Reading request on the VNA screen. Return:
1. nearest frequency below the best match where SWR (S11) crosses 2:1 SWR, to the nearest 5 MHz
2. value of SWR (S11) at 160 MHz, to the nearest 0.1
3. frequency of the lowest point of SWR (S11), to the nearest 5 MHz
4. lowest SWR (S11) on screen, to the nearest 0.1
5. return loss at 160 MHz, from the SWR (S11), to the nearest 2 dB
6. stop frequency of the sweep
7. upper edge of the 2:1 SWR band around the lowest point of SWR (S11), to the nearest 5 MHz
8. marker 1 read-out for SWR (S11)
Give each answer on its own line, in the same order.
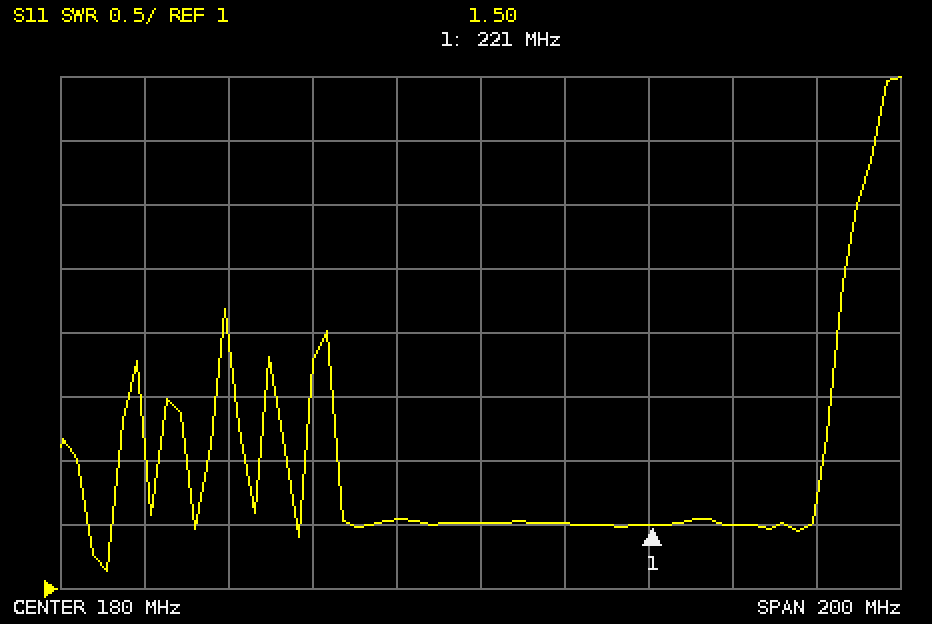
85 MHz
1.5
90 MHz
1.1
14 dB
280 MHz
95 MHz
1.50
